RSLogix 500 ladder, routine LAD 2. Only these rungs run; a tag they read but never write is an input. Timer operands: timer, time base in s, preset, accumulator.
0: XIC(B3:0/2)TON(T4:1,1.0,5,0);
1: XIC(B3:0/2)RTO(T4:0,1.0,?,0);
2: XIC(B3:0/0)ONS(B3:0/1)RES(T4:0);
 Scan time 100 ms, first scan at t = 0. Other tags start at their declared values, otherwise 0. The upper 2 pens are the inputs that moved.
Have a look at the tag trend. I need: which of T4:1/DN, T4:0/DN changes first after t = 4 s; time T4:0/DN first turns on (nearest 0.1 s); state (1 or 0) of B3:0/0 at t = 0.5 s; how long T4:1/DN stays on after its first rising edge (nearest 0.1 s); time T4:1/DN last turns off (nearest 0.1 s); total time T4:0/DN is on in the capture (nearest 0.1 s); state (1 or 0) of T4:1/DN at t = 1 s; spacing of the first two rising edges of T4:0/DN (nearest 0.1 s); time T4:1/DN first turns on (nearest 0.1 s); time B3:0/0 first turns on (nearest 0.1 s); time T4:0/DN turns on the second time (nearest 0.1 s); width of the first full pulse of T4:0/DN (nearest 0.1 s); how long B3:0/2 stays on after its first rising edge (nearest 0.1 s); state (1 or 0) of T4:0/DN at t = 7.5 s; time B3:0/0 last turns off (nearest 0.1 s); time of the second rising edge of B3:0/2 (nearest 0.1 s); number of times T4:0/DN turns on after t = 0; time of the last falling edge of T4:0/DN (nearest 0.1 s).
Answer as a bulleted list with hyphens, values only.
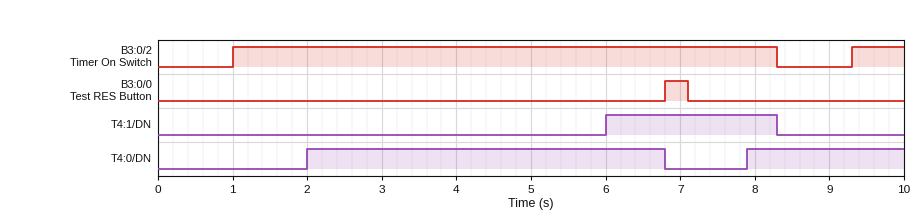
- T4:1/DN
- 2.0 s
- 0
- 2.3 s
- 8.3 s
- 6.9 s
- 0
- 5.9 s
- 6.0 s
- 6.8 s
- 7.9 s
- 4.8 s
- 7.3 s
- 0
- 7.1 s
- 9.3 s
- 2
- 6.8 s
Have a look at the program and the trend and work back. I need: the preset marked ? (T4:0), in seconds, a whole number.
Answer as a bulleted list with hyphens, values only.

- 1 s
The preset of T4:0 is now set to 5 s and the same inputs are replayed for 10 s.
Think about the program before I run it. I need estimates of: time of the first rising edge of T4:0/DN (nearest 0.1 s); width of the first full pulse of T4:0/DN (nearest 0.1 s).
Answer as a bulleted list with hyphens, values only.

- 6.0 s
- 0.8 s
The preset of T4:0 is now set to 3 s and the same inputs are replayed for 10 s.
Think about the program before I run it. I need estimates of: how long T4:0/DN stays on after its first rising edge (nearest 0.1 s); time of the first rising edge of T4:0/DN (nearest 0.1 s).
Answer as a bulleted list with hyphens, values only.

- 2.8 s
- 4.0 s
